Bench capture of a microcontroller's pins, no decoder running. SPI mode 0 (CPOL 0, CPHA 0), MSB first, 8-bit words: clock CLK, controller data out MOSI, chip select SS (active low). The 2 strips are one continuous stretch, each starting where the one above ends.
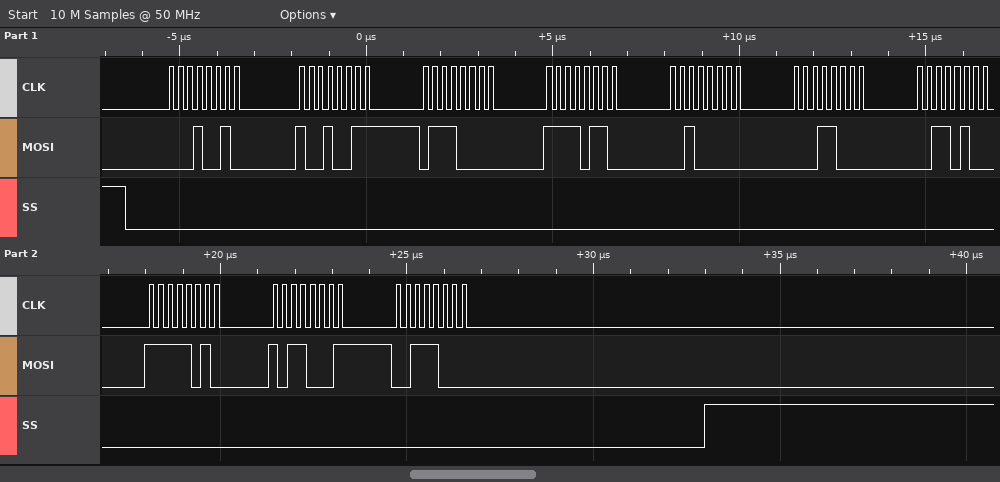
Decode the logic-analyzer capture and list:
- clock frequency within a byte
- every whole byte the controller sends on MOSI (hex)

4 MHz
0x12 0x93 0x70 0xF6 0x20 0x18 0x34 0xFA 0xB1 0x38
